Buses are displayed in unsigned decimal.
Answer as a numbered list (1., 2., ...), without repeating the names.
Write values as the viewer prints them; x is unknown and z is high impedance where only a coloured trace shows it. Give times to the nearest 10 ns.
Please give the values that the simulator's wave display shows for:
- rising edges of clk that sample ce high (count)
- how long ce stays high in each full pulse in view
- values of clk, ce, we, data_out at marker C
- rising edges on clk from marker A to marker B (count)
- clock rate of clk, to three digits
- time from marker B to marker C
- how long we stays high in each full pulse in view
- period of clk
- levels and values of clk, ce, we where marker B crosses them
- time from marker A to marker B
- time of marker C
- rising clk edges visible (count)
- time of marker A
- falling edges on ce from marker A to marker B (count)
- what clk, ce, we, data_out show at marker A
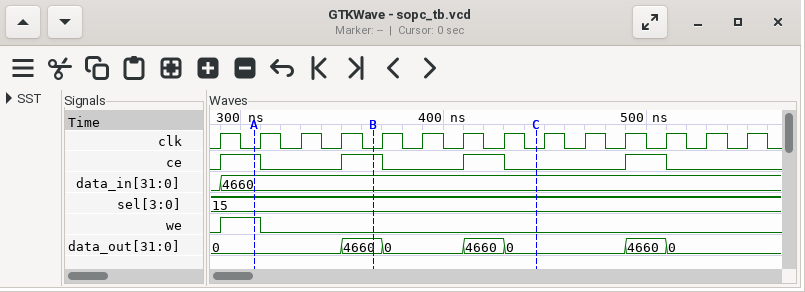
1. 4
2. 20 ns, 20 ns, 20 ns, 20 ns
3. clk=0, ce=0, we=0, data_out=0
4. 3
5. 50.0 MHz
6. 80 ns
7. 20 ns
8. 20 ns
9. clk=0, ce=1, we=0
10. 60 ns
11. 450 ns
12. 14
13. 310 ns
14. 1
15. clk=0, ce=1, we=1, data_out=0
